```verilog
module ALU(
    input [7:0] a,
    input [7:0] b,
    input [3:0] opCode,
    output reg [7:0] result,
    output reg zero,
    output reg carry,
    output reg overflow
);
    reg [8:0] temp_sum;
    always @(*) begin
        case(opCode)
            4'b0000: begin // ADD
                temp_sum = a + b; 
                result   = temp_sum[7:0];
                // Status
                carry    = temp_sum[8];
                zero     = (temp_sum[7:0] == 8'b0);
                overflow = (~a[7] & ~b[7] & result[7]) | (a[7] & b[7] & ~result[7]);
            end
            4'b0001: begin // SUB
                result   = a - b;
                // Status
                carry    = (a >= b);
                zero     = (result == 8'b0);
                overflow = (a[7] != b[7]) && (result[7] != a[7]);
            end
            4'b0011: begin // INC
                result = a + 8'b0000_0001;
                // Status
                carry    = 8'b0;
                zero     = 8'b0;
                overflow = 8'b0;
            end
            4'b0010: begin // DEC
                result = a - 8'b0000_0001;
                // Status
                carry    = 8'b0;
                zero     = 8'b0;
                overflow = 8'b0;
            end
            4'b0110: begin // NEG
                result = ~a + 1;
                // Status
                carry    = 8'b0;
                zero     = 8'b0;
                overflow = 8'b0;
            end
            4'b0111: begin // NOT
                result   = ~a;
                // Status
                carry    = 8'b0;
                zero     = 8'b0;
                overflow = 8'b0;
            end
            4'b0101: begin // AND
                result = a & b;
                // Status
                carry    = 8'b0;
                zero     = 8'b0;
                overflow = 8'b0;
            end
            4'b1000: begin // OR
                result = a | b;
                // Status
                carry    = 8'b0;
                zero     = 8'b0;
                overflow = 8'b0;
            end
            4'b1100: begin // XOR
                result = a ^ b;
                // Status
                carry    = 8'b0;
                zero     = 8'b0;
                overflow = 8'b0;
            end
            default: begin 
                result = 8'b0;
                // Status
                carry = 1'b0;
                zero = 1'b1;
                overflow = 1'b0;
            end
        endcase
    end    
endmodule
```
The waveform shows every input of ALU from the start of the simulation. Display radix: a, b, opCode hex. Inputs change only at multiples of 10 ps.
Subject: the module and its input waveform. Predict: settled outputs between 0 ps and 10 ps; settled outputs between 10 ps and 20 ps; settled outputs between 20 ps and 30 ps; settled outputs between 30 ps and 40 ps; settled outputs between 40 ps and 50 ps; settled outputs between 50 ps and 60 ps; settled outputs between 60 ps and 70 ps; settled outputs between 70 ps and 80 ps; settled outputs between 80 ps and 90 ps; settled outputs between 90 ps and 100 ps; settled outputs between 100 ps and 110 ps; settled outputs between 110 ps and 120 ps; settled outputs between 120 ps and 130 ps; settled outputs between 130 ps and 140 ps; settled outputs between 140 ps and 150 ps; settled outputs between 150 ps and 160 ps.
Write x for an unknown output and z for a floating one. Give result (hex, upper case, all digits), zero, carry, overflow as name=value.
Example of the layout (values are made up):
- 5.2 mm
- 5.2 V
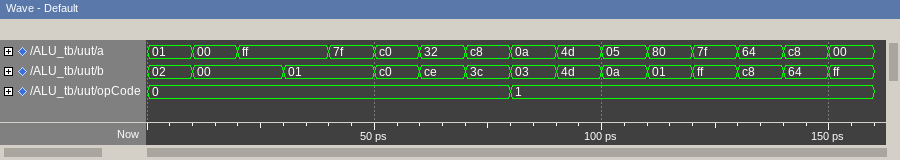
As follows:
- result=03, zero=0, carry=0, overflow=0
- result=00, zero=1, carry=0, overflow=0
- result=FF, zero=0, carry=0, overflow=0
- result=00, zero=1, carry=1, overflow=0
- result=80, zero=0, carry=0, overflow=1
- result=80, zero=0, carry=1, overflow=0
- result=00, zero=1, carry=1, overflow=0
- result=04, zero=0, carry=1, overflow=0
- result=07, zero=0, carry=1, overflow=0
- result=00, zero=1, carry=1, overflow=0
- result=FB, zero=0, carry=0, overflow=0
- result=7F, zero=0, carry=1, overflow=1
- result=80, zero=0, carry=0, overflow=1
- result=9C, zero=0, carry=0, overflow=1
- result=64, zero=0, carry=1, overflow=1
- result=01, zero=0, carry=0, overflow=0
